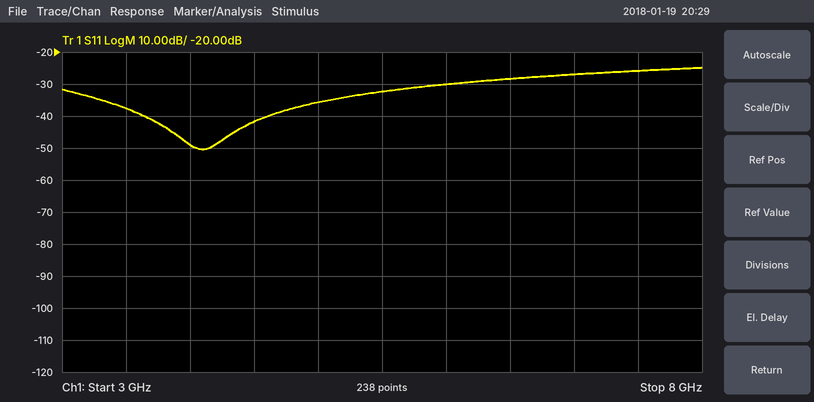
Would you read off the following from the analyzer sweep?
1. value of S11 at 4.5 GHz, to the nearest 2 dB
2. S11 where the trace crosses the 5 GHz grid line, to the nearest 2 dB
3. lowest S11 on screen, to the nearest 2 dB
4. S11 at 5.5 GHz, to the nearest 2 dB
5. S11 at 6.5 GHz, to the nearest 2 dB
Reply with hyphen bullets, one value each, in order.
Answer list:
- -42 dB
- -36 dB
- -50 dB
- -32 dB
- -28 dB
